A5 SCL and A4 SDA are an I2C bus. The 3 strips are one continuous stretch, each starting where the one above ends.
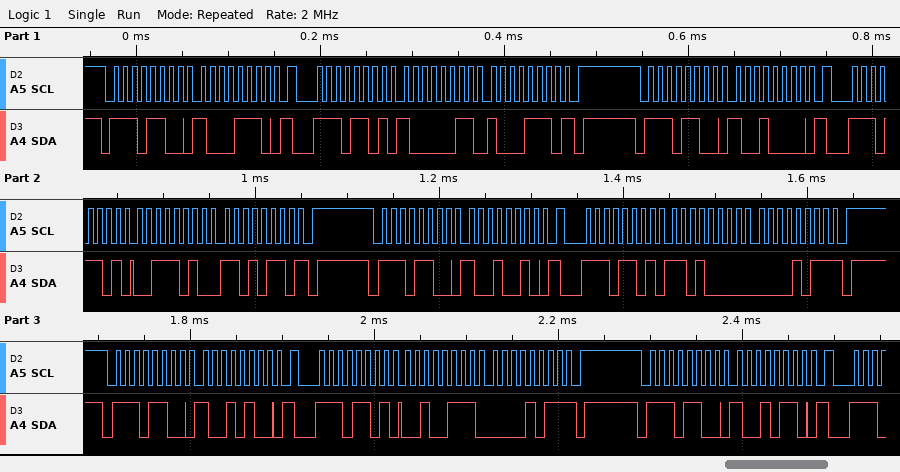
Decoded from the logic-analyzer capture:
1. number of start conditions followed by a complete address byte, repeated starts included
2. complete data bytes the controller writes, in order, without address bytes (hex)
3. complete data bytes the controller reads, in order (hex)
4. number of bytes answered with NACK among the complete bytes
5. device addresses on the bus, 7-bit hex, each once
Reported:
9
8E 90 92 94 96
83 8E 3A D6 D0 0B 27 0B
4
0x76
